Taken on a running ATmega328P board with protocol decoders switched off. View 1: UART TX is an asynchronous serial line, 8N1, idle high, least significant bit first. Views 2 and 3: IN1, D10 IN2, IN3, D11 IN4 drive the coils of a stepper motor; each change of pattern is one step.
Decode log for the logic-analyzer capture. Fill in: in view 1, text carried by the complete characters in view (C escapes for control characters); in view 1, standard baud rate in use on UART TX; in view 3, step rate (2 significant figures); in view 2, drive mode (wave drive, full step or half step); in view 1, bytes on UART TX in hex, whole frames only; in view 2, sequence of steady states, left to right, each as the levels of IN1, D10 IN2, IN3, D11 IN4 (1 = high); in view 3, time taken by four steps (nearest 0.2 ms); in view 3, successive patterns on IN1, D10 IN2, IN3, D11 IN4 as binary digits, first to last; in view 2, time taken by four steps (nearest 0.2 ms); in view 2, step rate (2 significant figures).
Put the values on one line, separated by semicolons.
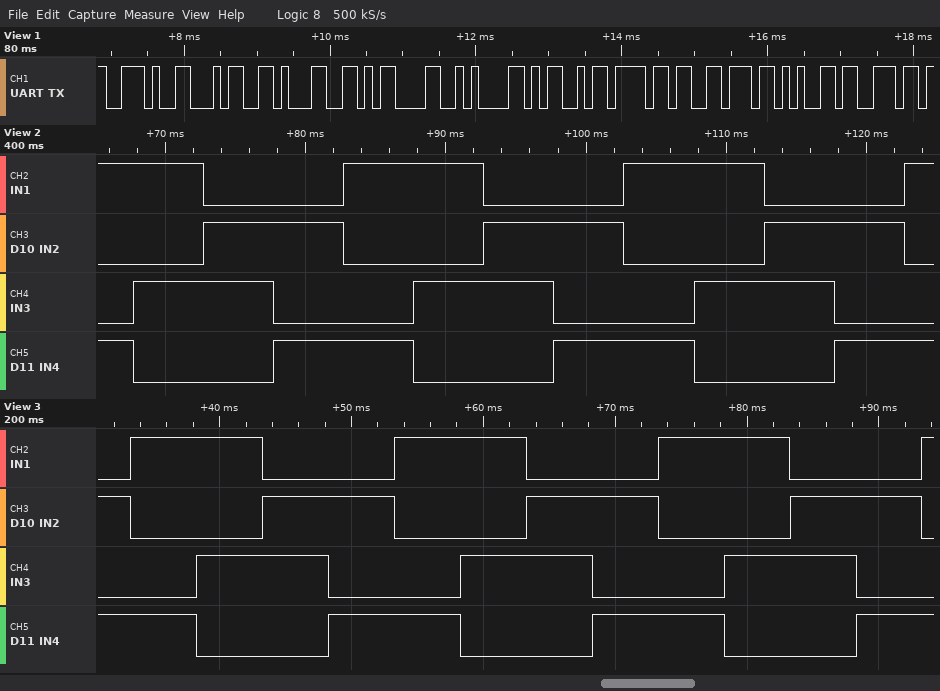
".41\r\nMoven"; 9600 baud; 200 steps/s; full step; 2E 34 31 0D 0A 4D 6F 76 65 6E; 1001 1010 0110 0101 1001 1010 0110 0101 1001 1010 0110 0101 1001; 20.0 ms; 0101 1001 1010 0110 0101 1001 1010 0110 0101 1001 1010 0110 0101 1001; 20.0 ms; 200 steps/s
